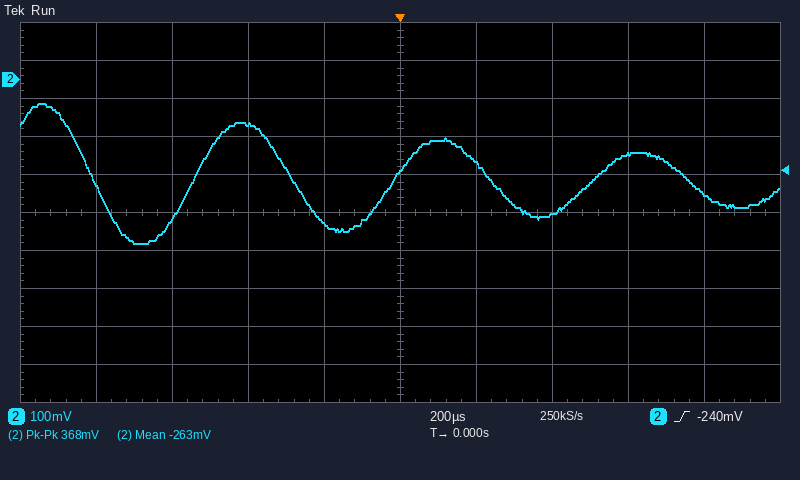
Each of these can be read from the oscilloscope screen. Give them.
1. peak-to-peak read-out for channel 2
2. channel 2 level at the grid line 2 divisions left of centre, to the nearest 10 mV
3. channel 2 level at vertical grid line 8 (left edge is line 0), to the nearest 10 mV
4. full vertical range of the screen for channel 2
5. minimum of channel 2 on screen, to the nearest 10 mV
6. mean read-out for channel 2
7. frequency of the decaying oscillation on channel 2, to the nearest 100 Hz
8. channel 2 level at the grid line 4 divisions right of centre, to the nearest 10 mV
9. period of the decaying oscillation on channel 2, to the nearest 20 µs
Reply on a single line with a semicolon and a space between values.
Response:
368 mV; -120 mV; -200 mV; 1 V; -430 mV; -263 mV; 1.9 kHz; -300 mV; 520 µs
